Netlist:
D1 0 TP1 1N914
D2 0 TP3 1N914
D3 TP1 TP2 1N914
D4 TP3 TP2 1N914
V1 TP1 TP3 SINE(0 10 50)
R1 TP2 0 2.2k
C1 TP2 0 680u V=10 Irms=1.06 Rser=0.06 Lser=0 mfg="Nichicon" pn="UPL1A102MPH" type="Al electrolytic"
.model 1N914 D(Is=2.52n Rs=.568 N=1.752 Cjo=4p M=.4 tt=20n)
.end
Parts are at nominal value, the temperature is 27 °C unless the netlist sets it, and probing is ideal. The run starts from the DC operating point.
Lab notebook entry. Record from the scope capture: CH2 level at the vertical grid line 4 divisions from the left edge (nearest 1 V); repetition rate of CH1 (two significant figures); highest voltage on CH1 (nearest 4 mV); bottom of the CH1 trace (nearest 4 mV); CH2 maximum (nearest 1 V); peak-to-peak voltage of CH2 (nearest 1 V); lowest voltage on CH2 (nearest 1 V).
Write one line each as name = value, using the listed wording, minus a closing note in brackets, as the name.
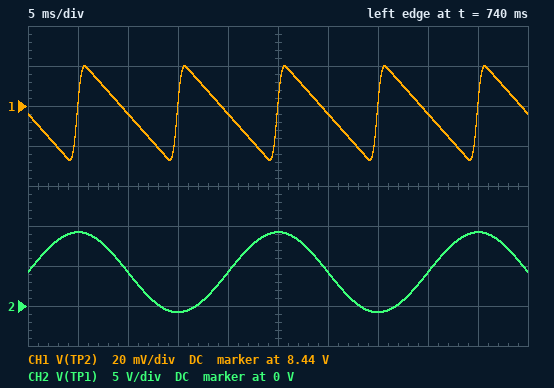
CH2 level at the vertical grid line 4 divisions from the left edge = 4 V
repetition rate of CH1 = 100 Hz
highest voltage on CH1 = 8.460 V
bottom of the CH1 trace = 8.412 V
CH2 maximum = 9 V
peak-to-peak voltage of CH2 = 10 V
lowest voltage on CH2 = -1 V
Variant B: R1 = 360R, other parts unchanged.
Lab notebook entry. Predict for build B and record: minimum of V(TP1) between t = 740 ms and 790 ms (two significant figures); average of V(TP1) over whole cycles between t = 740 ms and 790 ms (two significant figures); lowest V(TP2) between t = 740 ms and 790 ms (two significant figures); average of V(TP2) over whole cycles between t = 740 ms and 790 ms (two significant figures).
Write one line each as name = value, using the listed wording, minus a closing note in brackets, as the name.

minimum of V(TP1) between t = 740 ms and 790 ms = -930 mV
average of V(TP1) over whole cycles between t = 740 ms and 790 ms = 4.1 V
lowest V(TP2) between t = 740 ms and 790 ms = 8.0 V
average of V(TP2) over whole cycles between t = 740 ms and 790 ms = 8.1 V
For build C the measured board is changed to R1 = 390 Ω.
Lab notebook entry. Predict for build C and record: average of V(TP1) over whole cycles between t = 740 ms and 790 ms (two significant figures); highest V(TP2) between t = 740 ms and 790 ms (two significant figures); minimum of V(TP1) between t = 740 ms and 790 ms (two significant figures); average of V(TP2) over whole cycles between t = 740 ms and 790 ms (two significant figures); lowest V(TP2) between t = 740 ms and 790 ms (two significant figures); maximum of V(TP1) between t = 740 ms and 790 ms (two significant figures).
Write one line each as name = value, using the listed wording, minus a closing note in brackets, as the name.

average of V(TP1) over whole cycles between t = 740 ms and 790 ms = 4.1 V
highest V(TP2) between t = 740 ms and 790 ms = 8.3 V
minimum of V(TP1) between t = 740 ms and 790 ms = -920 mV
average of V(TP2) over whole cycles between t = 740 ms and 790 ms = 8.1 V
lowest V(TP2) between t = 740 ms and 790 ms = 8.0 V
maximum of V(TP1) between t = 740 ms and 790 ms = 9.1 V
